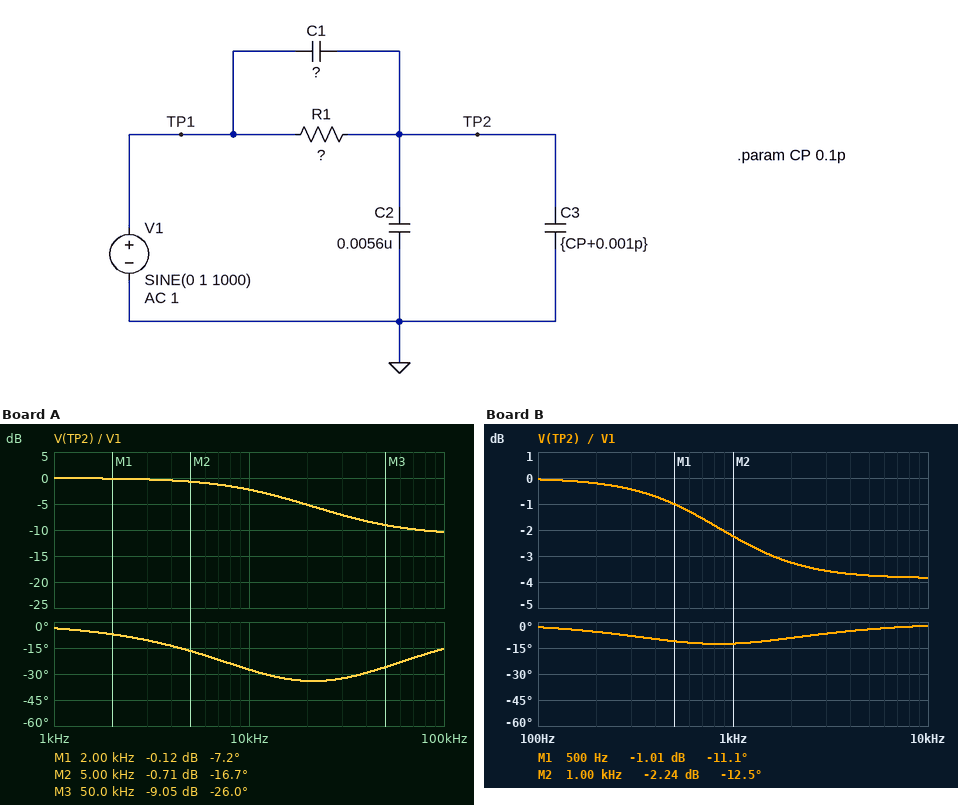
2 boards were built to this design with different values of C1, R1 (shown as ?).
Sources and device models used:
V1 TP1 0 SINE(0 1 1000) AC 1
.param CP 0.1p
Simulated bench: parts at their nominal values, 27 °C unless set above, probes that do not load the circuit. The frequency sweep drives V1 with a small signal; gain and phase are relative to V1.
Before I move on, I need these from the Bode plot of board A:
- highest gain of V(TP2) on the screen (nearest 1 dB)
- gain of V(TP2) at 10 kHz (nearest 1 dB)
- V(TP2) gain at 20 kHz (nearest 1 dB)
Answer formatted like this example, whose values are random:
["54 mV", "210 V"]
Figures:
["0 dB", "-2 dB", "-5 dB"]
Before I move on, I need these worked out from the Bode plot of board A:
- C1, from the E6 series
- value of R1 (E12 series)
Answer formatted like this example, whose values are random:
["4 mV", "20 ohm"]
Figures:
["2.2 nF", "1.8 kΩ"]
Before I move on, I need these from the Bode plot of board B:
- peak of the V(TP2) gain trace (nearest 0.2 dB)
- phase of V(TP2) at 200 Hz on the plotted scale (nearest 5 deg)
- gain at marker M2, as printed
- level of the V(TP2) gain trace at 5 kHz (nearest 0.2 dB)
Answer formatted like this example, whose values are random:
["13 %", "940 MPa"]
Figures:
["0 dB", "-5 deg", "-2.24 dB", "-3.8 dB"]
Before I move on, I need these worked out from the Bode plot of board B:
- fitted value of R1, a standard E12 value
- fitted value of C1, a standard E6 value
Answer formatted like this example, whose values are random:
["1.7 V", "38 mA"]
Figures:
["15 kΩ", "10 nF"]
